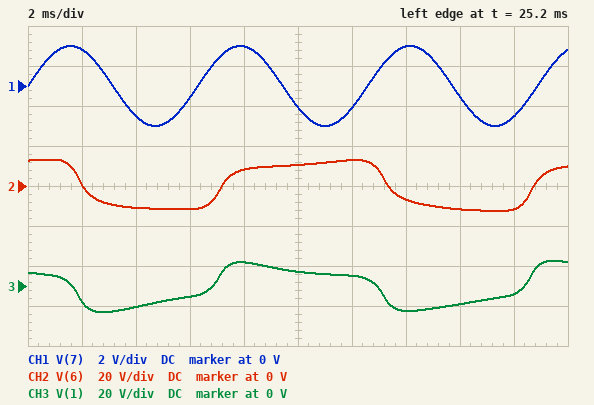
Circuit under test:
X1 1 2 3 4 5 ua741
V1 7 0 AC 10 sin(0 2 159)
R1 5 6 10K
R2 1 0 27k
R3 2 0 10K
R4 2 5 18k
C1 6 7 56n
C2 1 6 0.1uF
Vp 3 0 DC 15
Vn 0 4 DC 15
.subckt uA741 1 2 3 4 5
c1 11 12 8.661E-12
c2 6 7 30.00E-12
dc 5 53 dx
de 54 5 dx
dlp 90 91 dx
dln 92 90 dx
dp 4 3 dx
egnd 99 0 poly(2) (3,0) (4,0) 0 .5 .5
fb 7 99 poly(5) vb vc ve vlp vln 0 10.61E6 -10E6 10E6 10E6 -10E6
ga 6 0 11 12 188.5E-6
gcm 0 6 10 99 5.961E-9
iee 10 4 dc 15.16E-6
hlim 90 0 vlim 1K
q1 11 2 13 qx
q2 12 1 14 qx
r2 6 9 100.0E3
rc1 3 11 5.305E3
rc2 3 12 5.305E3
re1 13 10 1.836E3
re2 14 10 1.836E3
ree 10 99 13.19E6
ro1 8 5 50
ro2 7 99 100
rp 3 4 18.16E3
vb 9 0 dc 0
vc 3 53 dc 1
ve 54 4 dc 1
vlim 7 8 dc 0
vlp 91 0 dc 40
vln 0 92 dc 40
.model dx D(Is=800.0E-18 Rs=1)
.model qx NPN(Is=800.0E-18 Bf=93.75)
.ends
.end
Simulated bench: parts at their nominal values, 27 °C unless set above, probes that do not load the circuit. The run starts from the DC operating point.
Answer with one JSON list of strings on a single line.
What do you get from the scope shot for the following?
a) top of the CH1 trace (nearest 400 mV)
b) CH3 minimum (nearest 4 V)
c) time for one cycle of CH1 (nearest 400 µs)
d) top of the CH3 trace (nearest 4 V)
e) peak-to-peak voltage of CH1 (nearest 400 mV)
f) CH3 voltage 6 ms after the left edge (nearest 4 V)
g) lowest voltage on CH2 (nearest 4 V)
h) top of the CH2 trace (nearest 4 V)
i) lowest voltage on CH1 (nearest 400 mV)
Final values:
["2.0 V", "-12 V", "6.4 ms", "12 V", "4.0 V", "-4 V", "-12 V", "12 V", "-2.0 V"]
